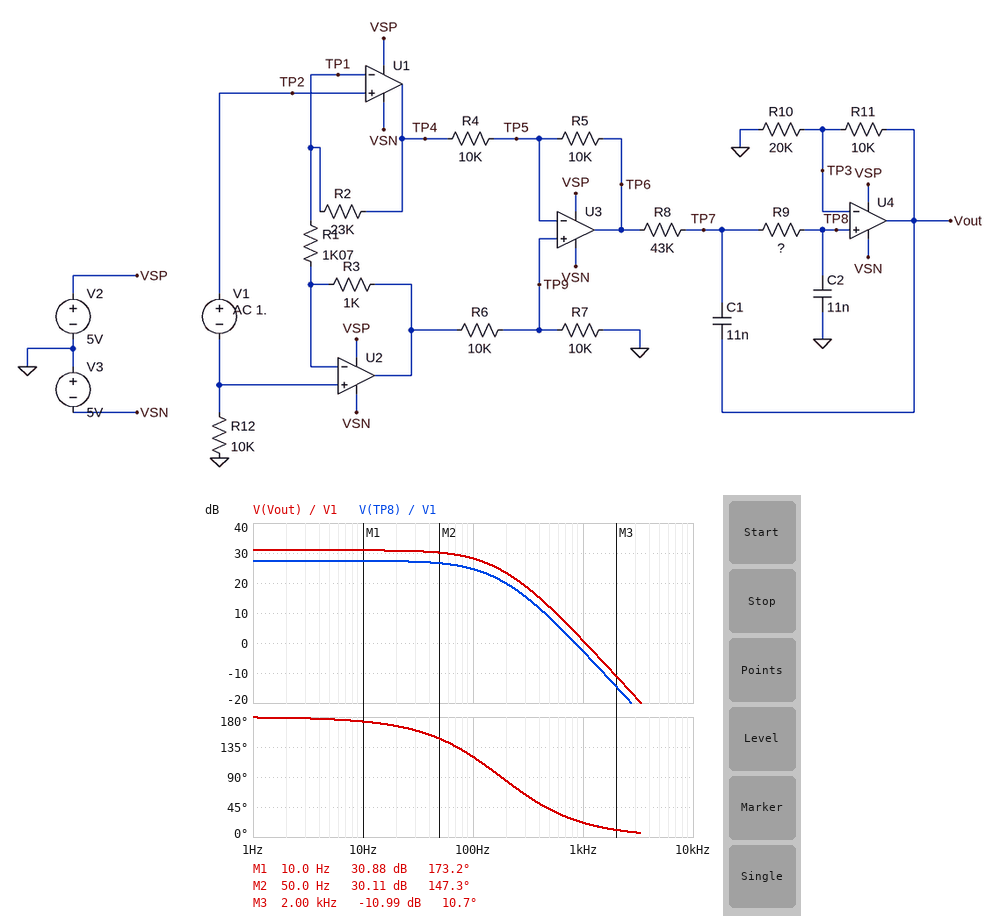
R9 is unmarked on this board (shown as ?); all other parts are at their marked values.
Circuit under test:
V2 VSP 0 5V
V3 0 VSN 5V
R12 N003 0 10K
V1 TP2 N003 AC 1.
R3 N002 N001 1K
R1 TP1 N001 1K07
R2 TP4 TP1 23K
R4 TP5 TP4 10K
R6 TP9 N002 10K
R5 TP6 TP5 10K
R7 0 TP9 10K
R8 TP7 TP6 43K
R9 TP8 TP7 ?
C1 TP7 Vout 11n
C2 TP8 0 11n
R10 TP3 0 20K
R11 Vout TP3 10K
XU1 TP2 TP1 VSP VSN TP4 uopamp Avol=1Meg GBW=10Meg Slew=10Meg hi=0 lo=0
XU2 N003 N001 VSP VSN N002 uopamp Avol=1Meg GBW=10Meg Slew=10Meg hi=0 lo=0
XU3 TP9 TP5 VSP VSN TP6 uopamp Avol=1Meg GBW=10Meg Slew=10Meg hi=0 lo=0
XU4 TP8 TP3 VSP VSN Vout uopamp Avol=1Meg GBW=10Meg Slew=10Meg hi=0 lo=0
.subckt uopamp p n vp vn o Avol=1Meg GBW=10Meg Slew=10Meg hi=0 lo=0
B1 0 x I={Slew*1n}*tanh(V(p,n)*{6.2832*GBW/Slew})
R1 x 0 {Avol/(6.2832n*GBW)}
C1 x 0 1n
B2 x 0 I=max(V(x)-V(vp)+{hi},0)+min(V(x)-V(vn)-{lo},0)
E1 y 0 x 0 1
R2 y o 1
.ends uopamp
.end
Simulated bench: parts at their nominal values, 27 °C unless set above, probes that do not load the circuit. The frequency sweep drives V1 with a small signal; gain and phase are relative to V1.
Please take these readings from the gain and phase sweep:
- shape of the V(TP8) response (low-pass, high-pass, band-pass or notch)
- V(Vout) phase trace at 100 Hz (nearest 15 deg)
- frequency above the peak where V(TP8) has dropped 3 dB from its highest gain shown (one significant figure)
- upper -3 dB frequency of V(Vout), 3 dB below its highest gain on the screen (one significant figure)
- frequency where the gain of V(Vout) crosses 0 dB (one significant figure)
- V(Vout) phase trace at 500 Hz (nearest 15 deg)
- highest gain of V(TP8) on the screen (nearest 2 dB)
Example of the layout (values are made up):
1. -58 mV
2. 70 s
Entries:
1. low-pass
2. 120 deg
3. 100 Hz
4. 100 Hz
5. 1 kHz
6. 45 deg
7. 28 dB
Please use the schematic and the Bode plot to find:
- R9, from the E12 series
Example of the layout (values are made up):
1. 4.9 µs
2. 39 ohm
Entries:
1. 150 kΩ
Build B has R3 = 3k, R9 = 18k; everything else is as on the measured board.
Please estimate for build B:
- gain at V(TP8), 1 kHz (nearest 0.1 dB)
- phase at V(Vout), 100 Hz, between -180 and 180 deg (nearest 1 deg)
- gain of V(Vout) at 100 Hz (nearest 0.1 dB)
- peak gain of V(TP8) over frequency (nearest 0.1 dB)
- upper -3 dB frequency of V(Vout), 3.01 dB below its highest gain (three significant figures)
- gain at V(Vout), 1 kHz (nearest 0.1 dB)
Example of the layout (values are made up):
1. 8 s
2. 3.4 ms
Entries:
1. 16.4 dB
2. 164 deg
3. 31.6 dB
4. 28.1 dB
5. 518 Hz
6. 19.9 dB
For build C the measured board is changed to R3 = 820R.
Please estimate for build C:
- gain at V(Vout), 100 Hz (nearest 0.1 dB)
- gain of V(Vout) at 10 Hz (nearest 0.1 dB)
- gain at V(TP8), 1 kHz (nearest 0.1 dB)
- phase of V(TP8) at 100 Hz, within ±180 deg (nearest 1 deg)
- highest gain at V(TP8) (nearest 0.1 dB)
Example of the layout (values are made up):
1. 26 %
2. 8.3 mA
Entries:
1. 28.1 dB
2. 30.8 dB
3. -2.8 dB
4. 120 deg
5. 27.3 dB
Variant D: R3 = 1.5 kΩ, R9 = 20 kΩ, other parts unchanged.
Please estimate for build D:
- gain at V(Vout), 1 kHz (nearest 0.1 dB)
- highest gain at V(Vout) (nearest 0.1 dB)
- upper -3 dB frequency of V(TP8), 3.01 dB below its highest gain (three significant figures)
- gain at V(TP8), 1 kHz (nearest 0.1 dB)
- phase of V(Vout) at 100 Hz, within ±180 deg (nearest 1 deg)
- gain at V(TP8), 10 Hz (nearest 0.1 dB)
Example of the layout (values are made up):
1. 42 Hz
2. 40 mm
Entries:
1. 18.6 dB
2. 31.1 dB
3. 493 Hz
4. 15.0 dB
5. 163 deg
6. 27.6 dB
